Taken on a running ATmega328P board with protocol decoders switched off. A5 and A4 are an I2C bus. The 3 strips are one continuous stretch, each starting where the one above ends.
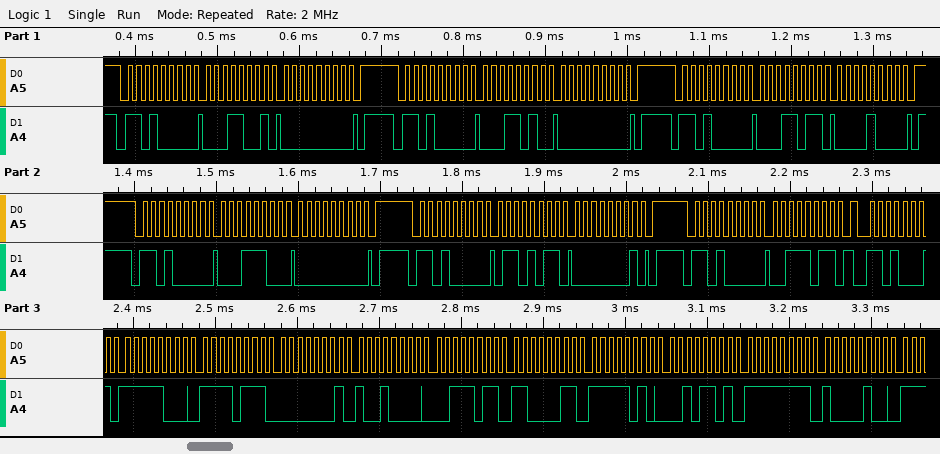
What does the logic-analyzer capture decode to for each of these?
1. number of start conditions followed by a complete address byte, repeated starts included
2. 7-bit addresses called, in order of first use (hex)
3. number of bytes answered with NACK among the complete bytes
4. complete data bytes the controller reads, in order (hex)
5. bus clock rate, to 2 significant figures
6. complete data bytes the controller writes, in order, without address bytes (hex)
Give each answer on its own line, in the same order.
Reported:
7
0x68
0
F8 F7 01 90 3B C3 FA 2D FF 84
100 kHz
19 00 1A 00 1B 08 1C 00 6B 01 3B
